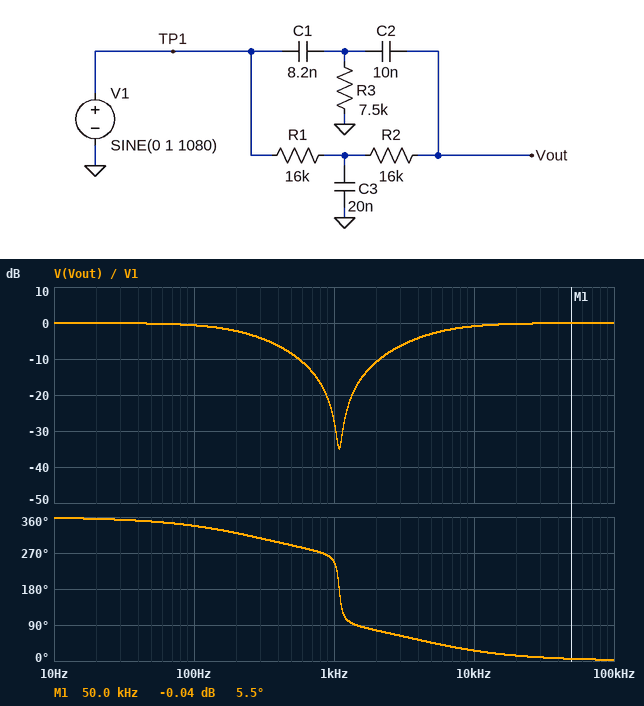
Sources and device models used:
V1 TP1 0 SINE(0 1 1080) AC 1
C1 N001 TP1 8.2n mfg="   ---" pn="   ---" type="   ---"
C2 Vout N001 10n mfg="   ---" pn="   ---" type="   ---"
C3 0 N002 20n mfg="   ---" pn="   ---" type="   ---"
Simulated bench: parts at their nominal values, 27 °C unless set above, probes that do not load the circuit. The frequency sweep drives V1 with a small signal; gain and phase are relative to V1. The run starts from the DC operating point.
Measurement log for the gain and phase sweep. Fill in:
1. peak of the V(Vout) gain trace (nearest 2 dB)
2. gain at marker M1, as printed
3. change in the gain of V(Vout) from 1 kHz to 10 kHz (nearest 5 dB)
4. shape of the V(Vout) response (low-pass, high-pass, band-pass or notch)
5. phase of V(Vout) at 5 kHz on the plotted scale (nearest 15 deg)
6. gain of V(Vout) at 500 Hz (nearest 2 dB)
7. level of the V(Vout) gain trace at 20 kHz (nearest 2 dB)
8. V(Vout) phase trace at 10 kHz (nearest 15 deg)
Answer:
0 dB
-0.04 dB
25 dB
notch
45 deg
-8 dB
0 dB
30 deg
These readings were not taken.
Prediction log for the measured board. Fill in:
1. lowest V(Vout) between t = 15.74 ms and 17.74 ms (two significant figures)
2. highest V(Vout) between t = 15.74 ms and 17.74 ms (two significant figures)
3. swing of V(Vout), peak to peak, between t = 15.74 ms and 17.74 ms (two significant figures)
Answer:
-18 mV
18 mV
36 mV
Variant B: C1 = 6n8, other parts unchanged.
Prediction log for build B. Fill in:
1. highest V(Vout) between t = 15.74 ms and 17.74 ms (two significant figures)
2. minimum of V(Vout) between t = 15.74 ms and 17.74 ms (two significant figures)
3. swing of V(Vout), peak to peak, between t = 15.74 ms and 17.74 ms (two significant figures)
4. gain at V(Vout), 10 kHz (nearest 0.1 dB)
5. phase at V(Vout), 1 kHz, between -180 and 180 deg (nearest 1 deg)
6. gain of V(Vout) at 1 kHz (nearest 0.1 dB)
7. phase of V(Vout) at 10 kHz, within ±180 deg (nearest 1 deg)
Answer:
43 mV
-43 mV
85 mV
-1.2 dB
-106 deg
-22.8 dB
30 deg
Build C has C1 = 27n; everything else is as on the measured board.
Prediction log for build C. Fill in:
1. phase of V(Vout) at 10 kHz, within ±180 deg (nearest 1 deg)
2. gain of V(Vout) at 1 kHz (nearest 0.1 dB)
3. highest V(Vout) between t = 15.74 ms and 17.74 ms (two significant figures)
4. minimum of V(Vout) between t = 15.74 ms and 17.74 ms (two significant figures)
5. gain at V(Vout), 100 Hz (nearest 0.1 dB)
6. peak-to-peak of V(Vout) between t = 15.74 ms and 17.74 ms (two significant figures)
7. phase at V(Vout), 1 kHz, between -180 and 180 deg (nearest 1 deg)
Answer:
12 deg
-12.9 dB
270 mV
-270 mV
-0.8 dB
540 mV
52 deg
